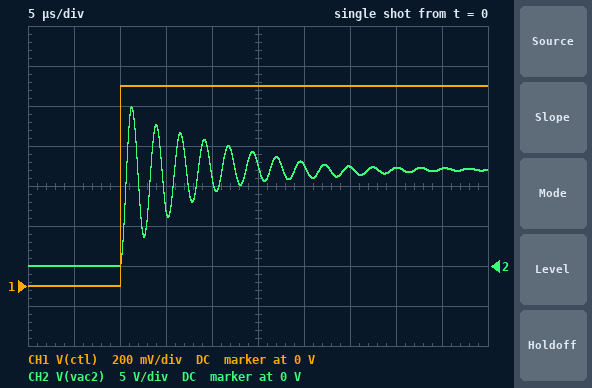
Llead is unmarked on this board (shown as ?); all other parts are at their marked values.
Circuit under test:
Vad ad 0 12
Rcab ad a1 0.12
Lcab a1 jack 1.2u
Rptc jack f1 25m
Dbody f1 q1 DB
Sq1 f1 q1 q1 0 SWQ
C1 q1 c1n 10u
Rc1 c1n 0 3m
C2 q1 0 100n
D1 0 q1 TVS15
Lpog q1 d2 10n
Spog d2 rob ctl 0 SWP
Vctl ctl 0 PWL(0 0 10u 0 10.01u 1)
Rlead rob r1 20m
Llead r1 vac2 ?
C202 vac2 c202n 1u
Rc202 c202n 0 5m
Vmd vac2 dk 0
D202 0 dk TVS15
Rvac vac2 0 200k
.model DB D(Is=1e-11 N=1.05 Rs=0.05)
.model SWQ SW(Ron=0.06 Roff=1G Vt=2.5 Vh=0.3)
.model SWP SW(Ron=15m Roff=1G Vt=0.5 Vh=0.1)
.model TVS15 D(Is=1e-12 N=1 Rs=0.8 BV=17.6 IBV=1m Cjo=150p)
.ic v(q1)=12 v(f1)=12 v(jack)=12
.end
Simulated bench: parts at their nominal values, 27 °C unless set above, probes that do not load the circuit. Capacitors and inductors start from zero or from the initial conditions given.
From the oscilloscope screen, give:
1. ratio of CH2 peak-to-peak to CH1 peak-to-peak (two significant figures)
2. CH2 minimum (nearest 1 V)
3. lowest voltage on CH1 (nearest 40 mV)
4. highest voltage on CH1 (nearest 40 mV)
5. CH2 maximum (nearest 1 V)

20
0 V
0 V
1.00 V
20 V
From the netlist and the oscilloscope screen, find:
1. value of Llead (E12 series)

180 nH
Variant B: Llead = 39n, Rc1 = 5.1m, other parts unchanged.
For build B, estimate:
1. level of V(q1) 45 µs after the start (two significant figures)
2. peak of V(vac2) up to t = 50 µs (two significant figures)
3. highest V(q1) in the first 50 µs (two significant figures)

12 V
19 V
12 V
